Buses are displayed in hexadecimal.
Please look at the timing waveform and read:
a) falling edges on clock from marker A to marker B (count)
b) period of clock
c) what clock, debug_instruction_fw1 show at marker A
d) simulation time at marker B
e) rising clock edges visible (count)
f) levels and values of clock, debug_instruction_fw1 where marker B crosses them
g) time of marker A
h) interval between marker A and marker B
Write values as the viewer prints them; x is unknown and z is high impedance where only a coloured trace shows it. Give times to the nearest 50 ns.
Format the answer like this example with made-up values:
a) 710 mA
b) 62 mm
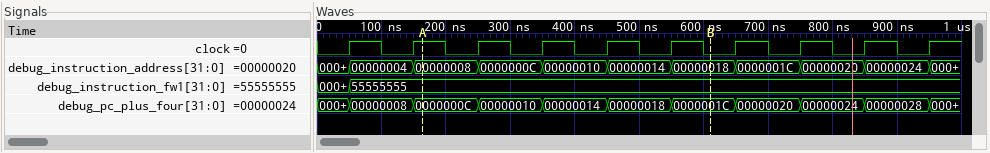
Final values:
a) 5
b) 100 ns
c) clock=1, debug_instruction_fw1=55555555
d) 600 ns
e) 10
f) clock=0, debug_instruction_fw1=55555555
g) 150 ns
h) 450 ns
